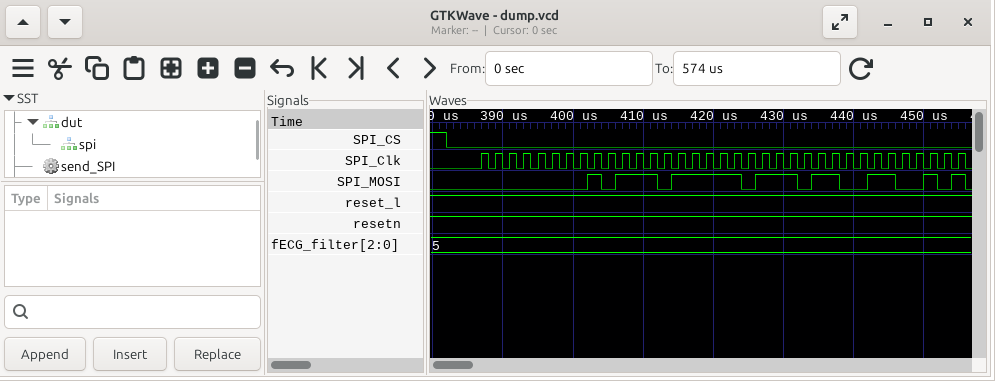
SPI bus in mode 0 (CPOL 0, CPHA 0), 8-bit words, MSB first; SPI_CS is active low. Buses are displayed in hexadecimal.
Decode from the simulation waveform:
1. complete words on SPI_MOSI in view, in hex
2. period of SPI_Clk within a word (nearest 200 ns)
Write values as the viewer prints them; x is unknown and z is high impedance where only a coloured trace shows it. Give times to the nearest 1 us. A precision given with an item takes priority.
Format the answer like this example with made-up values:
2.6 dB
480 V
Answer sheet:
00, BB, EE, CC
2000 ns
